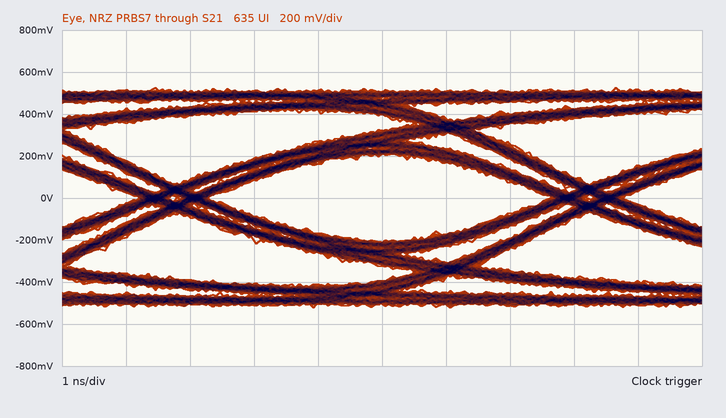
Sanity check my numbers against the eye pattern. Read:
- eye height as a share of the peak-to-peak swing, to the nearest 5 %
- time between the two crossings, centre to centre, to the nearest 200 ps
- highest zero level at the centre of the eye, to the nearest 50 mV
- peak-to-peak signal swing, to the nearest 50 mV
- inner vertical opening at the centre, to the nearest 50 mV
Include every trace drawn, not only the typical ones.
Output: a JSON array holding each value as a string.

["40 %", "6.4 ns", "-200 mV", "1.05 V", "400 mV"]
